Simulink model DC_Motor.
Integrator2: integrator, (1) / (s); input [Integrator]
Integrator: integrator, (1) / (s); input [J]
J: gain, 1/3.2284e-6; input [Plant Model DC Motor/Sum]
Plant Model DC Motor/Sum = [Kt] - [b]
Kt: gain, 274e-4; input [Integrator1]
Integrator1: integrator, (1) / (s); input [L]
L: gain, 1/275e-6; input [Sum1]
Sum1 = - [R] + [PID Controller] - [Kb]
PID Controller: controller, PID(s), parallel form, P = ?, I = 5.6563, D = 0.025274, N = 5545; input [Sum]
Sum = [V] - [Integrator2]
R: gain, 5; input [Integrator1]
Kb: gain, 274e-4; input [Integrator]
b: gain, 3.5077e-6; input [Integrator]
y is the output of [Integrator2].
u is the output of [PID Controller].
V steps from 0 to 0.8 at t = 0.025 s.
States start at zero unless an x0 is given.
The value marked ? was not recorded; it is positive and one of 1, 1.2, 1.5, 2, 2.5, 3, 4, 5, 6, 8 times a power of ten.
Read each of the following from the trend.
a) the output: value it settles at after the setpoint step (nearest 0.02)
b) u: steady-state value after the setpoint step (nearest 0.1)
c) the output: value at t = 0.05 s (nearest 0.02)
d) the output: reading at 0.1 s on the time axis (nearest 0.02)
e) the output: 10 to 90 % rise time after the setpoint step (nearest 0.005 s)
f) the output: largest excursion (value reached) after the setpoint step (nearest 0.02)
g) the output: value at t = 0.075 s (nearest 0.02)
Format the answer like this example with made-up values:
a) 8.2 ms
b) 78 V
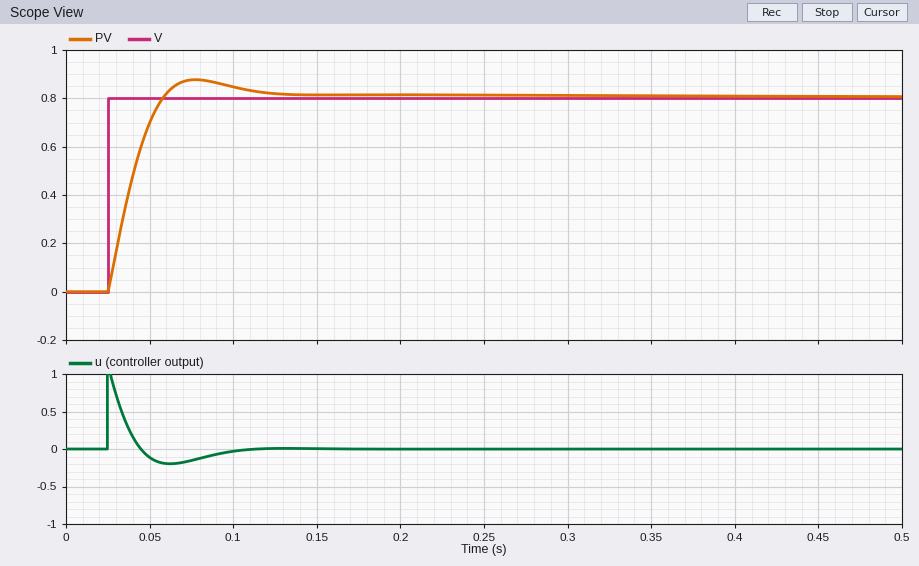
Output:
a) 0.80
b) 0.0
c) 0.70
d) 0.84
e) 0.025 s
f) 0.88
g) 0.88
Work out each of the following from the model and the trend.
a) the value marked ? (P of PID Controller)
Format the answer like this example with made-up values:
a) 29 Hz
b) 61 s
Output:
a) 2.5
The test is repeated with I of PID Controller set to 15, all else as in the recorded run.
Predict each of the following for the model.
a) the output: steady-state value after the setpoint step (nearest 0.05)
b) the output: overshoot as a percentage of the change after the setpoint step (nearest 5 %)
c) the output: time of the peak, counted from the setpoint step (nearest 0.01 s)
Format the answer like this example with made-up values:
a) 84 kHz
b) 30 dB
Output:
a) 0.80
b) 15 %
c) 0.05 s
